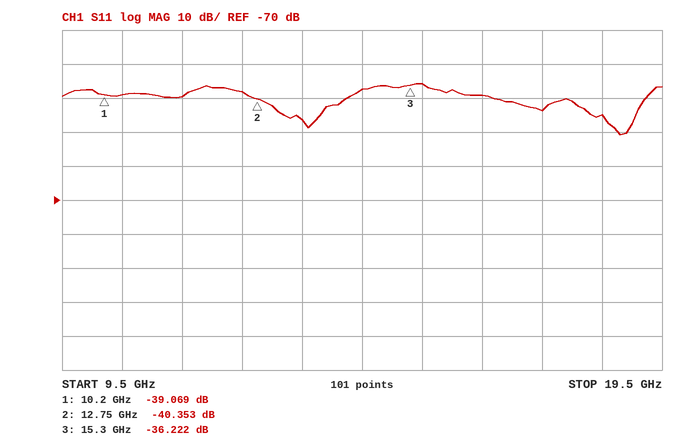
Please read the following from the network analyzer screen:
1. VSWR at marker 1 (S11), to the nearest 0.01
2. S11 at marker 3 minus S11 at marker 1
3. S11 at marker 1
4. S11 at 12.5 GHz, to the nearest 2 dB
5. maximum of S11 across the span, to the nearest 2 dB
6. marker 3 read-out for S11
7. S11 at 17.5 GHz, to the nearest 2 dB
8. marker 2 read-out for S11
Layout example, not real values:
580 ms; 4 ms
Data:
1.02; 2.847 dB; -39.069 dB; -38 dB; -36 dB; -36.222 dB; -44 dB; -40.353 dB
